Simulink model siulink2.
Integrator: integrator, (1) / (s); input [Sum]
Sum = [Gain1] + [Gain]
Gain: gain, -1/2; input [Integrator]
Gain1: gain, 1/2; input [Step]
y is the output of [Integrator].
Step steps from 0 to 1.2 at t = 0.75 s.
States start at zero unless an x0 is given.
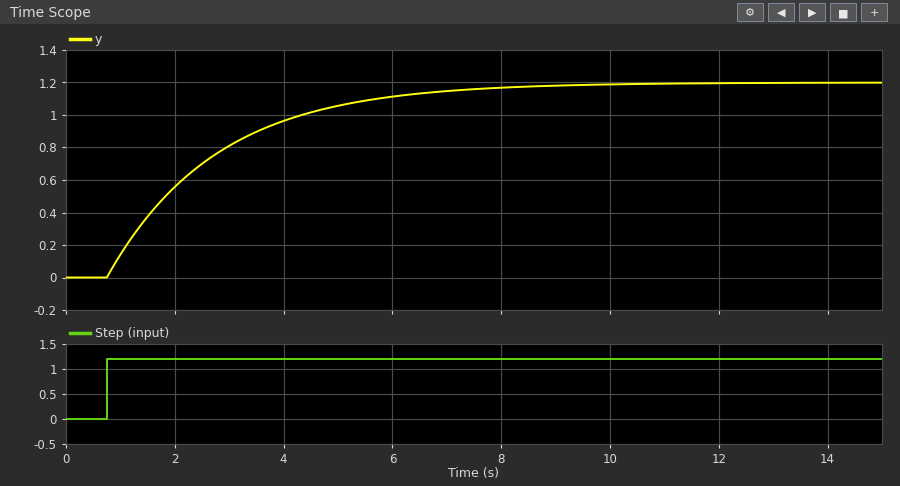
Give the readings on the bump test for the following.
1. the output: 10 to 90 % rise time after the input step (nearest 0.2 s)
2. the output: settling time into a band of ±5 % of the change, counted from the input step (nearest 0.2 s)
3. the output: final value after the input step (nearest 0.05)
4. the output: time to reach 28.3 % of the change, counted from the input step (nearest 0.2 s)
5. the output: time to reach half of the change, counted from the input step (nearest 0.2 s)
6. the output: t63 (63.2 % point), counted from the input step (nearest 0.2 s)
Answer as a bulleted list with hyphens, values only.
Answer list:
- 4.4 s
- 6.0 s
- 1.20
- 0.6 s
- 1.4 s
- 2.0 s
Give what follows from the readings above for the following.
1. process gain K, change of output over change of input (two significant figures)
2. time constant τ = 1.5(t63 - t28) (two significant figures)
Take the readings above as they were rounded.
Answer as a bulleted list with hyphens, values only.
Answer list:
- 1.0
- 2.1 s
